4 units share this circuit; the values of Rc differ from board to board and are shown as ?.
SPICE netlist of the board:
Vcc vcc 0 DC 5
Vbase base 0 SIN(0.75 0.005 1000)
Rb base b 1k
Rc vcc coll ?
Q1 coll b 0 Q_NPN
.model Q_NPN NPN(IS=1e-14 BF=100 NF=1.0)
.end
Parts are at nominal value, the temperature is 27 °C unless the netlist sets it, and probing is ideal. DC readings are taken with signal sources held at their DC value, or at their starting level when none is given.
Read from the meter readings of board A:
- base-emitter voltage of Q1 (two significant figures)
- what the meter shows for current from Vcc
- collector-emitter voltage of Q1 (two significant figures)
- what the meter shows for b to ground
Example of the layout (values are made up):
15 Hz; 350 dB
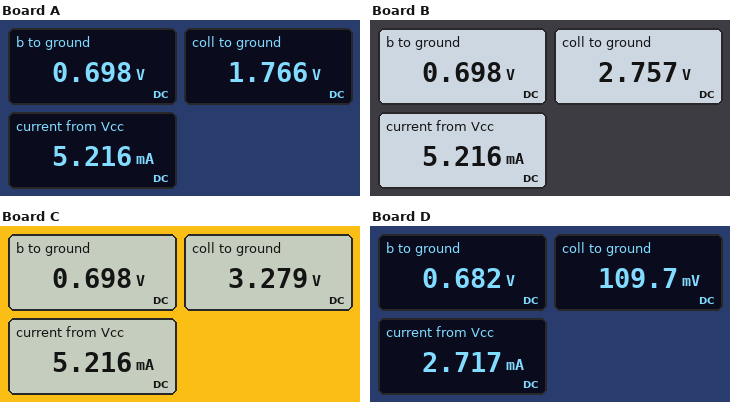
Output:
700 mV; 5.216 mA; 1.8 V; 0.698 V
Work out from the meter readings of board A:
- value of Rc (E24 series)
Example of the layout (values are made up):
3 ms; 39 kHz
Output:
620 Ω
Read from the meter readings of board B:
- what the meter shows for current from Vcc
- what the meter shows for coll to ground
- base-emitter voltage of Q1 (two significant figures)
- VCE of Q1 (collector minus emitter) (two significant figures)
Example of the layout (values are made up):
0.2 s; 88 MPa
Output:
5.216 mA; 2.757 V; 700 mV; 2.8 V
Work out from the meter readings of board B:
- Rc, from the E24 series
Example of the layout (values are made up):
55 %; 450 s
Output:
430 Ω
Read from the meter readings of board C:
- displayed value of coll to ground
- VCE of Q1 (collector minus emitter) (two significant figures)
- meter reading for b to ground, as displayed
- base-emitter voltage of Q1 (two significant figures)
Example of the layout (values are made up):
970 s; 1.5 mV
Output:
3.279 V; 3.3 V; 0.698 V; 700 mV
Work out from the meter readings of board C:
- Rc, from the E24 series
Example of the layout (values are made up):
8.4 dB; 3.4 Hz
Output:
330 Ω
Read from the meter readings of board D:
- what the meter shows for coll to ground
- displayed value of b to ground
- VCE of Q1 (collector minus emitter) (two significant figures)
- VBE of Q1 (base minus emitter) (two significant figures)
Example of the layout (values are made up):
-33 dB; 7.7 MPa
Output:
109.7 mV; 0.682 V; 110 mV; 680 mV
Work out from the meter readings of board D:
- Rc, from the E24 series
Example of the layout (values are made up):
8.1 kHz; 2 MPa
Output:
1.8 kΩ
